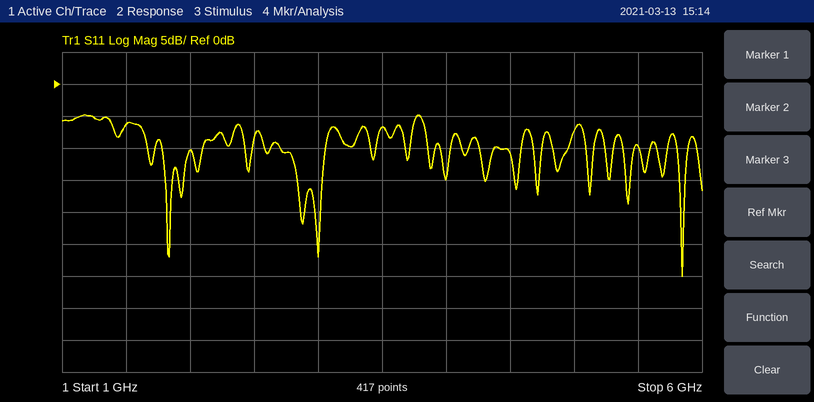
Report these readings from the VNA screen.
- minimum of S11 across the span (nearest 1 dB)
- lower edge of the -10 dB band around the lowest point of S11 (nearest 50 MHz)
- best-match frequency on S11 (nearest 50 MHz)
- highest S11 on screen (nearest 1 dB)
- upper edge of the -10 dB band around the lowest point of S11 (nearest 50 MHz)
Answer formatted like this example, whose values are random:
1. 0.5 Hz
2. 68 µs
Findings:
1. -30 dB
2. 5.80 GHz
3. 5.85 GHz
4. -5 dB
5. 5.90 GHz
